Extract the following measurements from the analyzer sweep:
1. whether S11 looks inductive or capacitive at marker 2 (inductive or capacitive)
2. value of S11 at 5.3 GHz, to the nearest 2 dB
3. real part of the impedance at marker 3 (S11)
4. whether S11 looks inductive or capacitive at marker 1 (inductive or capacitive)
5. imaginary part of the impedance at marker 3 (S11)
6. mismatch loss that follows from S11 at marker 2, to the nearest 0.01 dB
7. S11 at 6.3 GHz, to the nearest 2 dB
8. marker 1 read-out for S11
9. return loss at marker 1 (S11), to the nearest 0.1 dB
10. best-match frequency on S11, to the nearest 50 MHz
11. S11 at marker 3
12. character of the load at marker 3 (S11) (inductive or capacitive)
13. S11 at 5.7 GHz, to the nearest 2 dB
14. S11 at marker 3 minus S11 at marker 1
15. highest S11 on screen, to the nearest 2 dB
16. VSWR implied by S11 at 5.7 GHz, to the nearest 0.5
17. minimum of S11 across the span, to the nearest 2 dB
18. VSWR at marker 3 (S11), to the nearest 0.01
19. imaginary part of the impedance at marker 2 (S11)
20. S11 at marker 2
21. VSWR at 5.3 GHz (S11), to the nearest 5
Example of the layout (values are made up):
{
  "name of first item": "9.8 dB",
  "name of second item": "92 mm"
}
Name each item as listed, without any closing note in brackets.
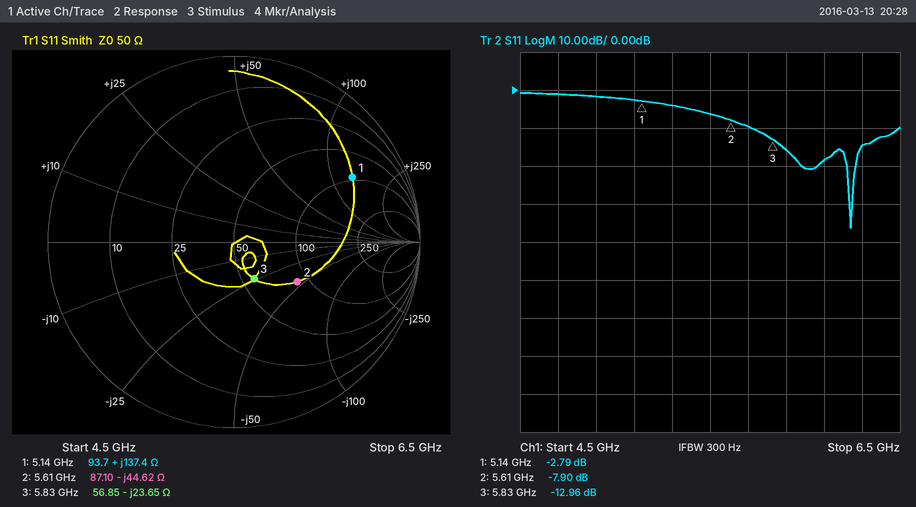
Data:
{
  "whether S11 looks inductive or capacitive at marker 2": "capacitive",
  "value of S11 at 5.3 GHz, to the nearest 2 dB": "-4 dB",
  "real part of the impedance at marker 3": "56.85 Ω",
  "whether S11 looks inductive or capacitive at marker 1": "inductive",
  "imaginary part of the impedance at marker 3": "-23.65 Ω",
  "mismatch loss that follows from S11 at marker 2, to the nearest 0.01 dB": "0.77 dB",
  "S11 at 6.3 GHz, to the nearest 2 dB": "-14 dB",
  "marker 1 read-out for S11": "-2.79 dB",
  "return loss at marker 1 (S11), to the nearest 0.1 dB": "2.8 dB",
  "best-match frequency on S11, to the nearest 50 MHz": "6.25 GHz",
  "S11 at marker 3": "-12.96 dB",
  "character of the load at marker 3 (S11)": "capacitive",
  "S11 at 5.7 GHz, to the nearest 2 dB": "-10 dB",
  "S11 at marker 3 minus S11 at marker 1": "-10.17 dB",
  "highest S11 on screen, to the nearest 2 dB": "0 dB",
  "VSWR implied by S11 at 5.7 GHz, to the nearest 0.5": "2.0",
  "minimum of S11 across the span, to the nearest 2 dB": "-36 dB",
  "VSWR at marker 3 (S11), to the nearest 0.01": "1.58",
  "imaginary part of the impedance at marker 2": "-44.62 Ω",
  "S11 at marker 2": "-7.90 dB",
  "VSWR at 5.3 GHz (S11), to the nearest 5": "5"
}
